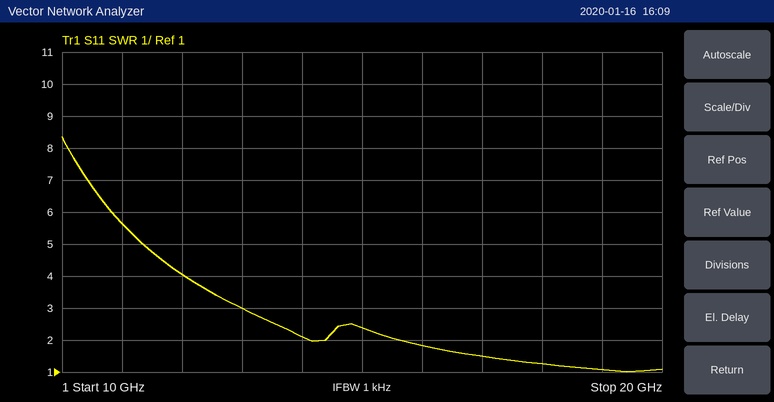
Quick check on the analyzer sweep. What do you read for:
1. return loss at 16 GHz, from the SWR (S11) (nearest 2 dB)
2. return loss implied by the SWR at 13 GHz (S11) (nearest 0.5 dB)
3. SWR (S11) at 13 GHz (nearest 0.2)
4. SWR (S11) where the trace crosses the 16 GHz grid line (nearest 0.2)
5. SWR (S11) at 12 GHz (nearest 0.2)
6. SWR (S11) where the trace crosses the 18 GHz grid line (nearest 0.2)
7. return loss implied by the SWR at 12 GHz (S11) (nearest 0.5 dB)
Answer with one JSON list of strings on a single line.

["10 dB", "6.0 dB", "3.0", "1.8", "4.0", "1.2", "4.5 dB"]
